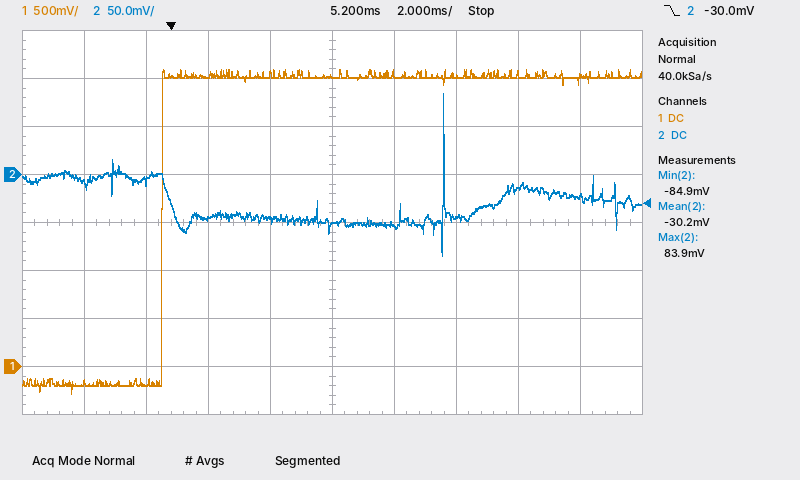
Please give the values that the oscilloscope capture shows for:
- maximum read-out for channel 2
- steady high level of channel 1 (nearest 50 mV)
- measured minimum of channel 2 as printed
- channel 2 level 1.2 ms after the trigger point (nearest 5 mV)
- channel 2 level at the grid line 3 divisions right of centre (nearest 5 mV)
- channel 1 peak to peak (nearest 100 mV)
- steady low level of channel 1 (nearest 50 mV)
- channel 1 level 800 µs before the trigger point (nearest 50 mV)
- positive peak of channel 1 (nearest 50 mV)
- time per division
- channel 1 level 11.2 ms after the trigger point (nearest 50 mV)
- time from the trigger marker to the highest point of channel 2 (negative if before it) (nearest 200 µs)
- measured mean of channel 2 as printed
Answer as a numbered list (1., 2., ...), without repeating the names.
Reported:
1. 83.9 mV
2. 3.00 V
3. -84.9 mV
4. -45 mV
5. -15 mV
6. 3.40 V
7. -200 mV
8. -150 mV
9. 3.10 V
10. 2 ms
11. 3.05 V
12. +8.8 ms
13. -30.2 mV
